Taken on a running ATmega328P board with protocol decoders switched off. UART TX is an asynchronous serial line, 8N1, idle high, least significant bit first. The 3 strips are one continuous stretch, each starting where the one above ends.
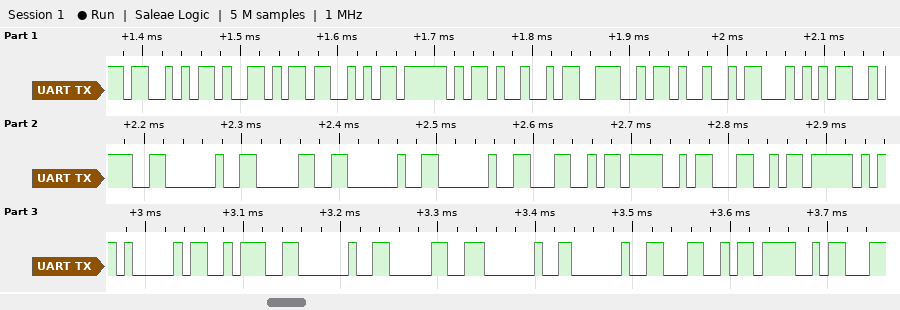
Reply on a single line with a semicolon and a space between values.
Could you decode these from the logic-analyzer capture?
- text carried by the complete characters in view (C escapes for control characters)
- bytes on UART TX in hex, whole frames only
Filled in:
"SYS_INIT: 0  LOL_A: 0  LO"; 0x53 0x59 0x53 0x5F 0x49 0x4E 0x49 0x54 0x3A 0x20 0x30 0x20 0x20 0x4C 0x4F 0x4C 0x5F 0x41 0x3A 0x20 0x30 0x20 0x20 0x4C 0x4F
